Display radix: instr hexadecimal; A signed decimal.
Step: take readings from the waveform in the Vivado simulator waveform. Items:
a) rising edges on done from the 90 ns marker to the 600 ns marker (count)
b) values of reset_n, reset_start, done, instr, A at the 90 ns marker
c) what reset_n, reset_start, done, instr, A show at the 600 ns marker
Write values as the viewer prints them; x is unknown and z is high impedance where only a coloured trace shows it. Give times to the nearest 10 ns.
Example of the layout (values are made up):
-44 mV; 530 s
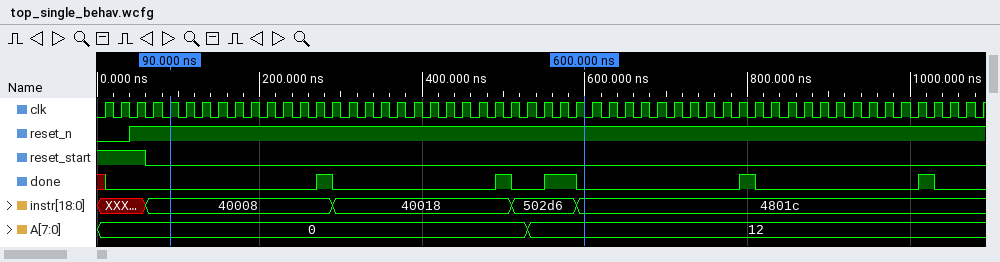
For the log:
3; reset_n=1, reset_start=0, done=0, instr=40008, A=0; reset_n=1, reset_start=0, done=0, instr=4801c, A=12
